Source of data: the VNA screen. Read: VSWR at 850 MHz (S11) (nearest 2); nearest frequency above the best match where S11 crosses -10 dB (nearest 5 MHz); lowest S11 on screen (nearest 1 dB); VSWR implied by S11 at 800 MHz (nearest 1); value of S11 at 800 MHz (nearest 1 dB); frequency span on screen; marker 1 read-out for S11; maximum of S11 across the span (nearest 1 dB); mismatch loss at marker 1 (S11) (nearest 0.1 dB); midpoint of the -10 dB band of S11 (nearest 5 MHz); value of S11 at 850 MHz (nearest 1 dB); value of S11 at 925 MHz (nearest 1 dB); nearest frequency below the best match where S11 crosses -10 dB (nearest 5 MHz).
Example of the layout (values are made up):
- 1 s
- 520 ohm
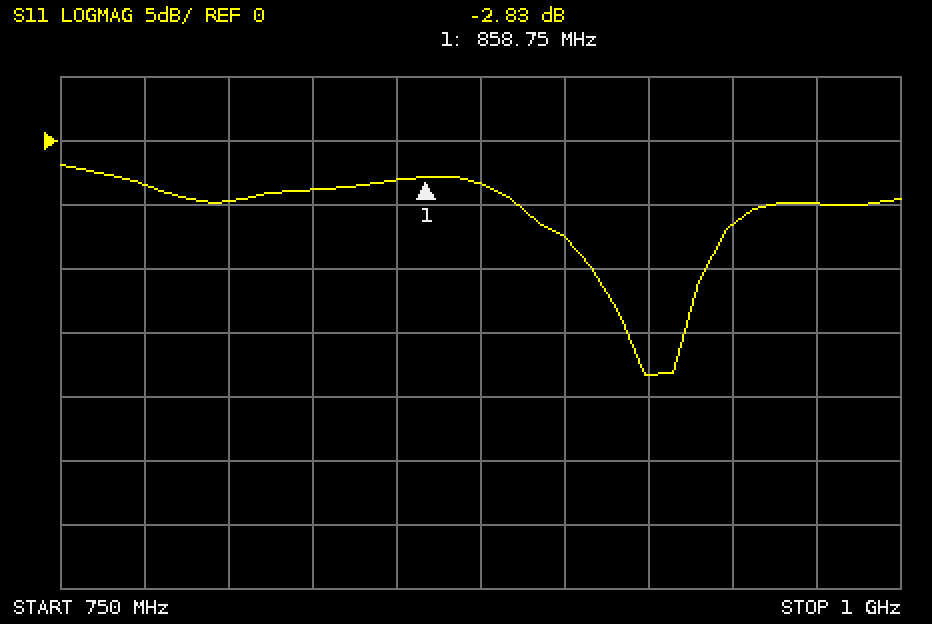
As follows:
- 6
- 940 MHz
- -18 dB
- 4
- -5 dB
- 250 MHz
- -2.83 dB
- -2 dB
- 3.2 dB
- 925 MHz
- -3 dB
- -18 dB
- 910 MHz
